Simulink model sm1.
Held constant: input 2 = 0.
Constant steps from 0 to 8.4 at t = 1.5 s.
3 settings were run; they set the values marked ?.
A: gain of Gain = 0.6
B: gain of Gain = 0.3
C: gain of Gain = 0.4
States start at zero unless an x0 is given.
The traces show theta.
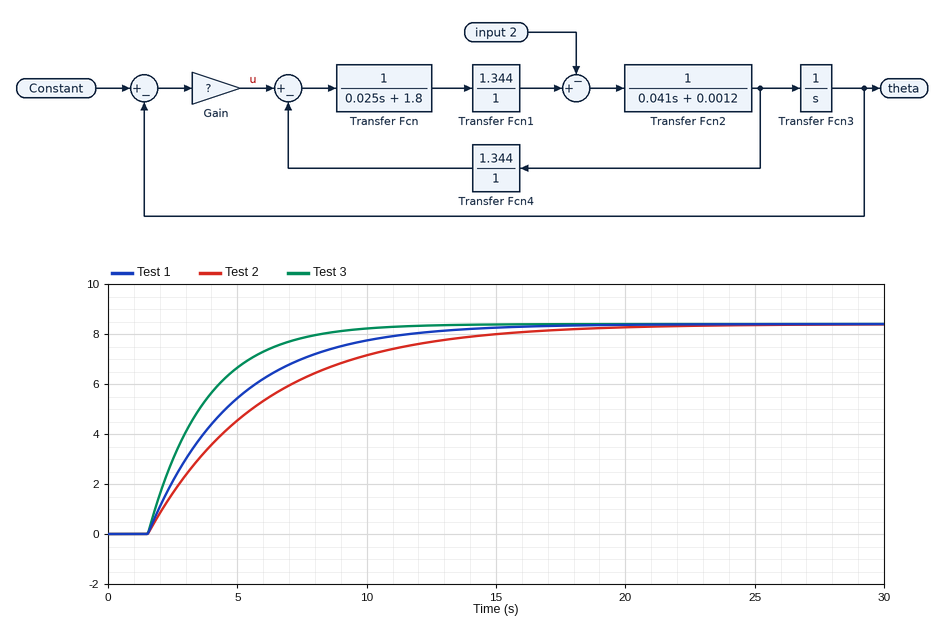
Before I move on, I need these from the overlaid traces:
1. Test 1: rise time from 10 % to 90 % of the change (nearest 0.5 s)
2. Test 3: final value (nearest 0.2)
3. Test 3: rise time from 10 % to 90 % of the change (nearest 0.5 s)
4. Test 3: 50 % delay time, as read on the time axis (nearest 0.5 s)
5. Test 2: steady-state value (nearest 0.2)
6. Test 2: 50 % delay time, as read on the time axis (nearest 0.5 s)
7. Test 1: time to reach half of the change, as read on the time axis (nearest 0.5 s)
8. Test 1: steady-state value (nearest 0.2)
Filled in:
7.5 s
8.4
5.0 s
3.0 s
8.4
4.5 s
4.0 s
8.4
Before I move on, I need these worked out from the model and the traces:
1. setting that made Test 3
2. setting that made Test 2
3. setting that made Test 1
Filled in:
A
B
C
